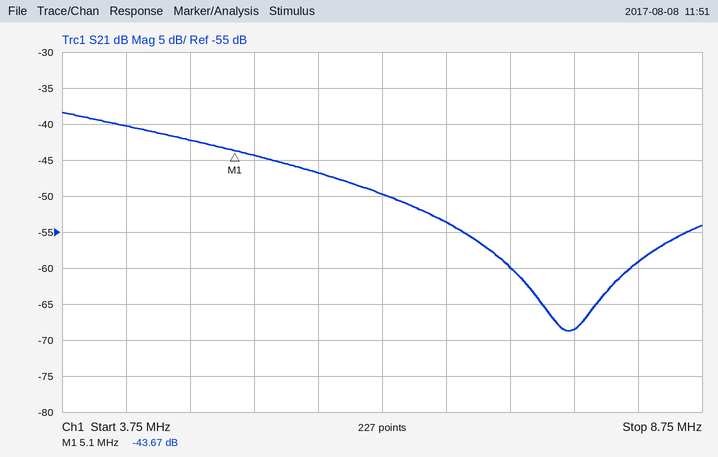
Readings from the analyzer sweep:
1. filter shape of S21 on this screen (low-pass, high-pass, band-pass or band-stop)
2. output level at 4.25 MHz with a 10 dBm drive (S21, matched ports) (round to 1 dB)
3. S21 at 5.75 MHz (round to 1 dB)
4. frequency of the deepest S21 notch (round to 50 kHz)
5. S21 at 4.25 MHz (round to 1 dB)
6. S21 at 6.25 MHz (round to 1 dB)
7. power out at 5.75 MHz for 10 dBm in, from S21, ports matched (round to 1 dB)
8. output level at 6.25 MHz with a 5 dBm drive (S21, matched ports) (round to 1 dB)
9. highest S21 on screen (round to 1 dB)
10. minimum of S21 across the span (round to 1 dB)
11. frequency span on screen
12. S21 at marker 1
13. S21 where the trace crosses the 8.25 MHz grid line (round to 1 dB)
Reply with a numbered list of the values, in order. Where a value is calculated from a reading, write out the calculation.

1. low-pass
2. 10 dBm + (-40 dB) = -30 dBm
3. -47 dB
4. 7.70 MHz
5. -40 dB
6. -50 dB
7. 10 dBm + (-47 dB) = -37 dBm
8. 5 dBm + (-50 dB) = -45 dBm
9. -38 dB
10. -69 dB
11. 5 MHz
12. -43.67 dB
13. -59 dB
